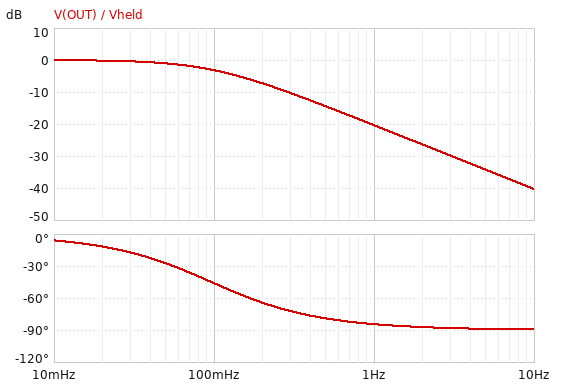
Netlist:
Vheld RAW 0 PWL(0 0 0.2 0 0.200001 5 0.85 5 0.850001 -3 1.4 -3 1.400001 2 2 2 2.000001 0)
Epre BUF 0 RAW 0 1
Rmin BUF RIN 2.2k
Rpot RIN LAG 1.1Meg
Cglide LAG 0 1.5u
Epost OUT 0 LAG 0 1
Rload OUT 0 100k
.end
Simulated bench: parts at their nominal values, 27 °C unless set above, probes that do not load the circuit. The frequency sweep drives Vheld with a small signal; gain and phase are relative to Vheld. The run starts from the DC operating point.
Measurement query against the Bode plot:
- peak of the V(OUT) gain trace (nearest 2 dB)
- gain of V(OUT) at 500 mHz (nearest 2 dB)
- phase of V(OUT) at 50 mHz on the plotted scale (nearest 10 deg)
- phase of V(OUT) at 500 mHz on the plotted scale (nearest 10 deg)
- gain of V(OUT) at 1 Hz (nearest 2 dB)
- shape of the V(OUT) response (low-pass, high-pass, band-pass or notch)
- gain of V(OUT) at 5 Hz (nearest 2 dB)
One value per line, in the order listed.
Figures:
0 dB
-14 dB
-30 deg
-80 deg
-20 dB
low-pass
-34 dB
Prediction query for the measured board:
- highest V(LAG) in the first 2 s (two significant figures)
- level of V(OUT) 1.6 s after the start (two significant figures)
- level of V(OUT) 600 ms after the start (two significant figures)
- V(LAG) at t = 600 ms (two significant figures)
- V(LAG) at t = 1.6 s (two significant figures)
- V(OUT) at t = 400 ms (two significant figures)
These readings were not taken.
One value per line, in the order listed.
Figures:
1.6 V
510 mV
1.1 V
1.1 V
510 mV
570 mV
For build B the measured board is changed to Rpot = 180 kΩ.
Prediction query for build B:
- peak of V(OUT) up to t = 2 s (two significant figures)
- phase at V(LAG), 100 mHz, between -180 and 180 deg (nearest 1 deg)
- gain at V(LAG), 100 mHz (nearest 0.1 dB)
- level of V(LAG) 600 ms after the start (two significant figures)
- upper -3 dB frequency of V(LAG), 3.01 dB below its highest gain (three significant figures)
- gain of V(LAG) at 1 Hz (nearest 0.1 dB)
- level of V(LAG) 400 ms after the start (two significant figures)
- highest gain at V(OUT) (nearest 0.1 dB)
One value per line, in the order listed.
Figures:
4.5 V
-10 deg
-0.1 dB
3.8 V
582 mHz
-6.0 dB
2.6 V
0 dB
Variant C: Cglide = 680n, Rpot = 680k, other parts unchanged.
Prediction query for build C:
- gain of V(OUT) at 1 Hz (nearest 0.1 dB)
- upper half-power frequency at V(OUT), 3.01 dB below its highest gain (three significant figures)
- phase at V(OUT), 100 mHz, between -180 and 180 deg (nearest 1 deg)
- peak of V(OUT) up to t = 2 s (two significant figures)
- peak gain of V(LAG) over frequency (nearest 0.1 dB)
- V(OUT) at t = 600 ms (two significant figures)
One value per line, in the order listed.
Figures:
-9.8 dB
343 mHz
-16 deg
3.8 V
0 dB
2.9 V
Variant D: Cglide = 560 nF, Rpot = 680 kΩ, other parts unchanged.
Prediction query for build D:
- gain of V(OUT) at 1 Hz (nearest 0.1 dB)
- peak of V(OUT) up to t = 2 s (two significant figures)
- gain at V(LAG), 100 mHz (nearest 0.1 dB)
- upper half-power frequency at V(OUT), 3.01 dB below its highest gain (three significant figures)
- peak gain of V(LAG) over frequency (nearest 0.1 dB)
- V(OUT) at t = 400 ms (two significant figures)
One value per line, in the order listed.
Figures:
-8.3 dB
4.1 V
-0.2 dB
417 mHz
0 dB
2.0 V
